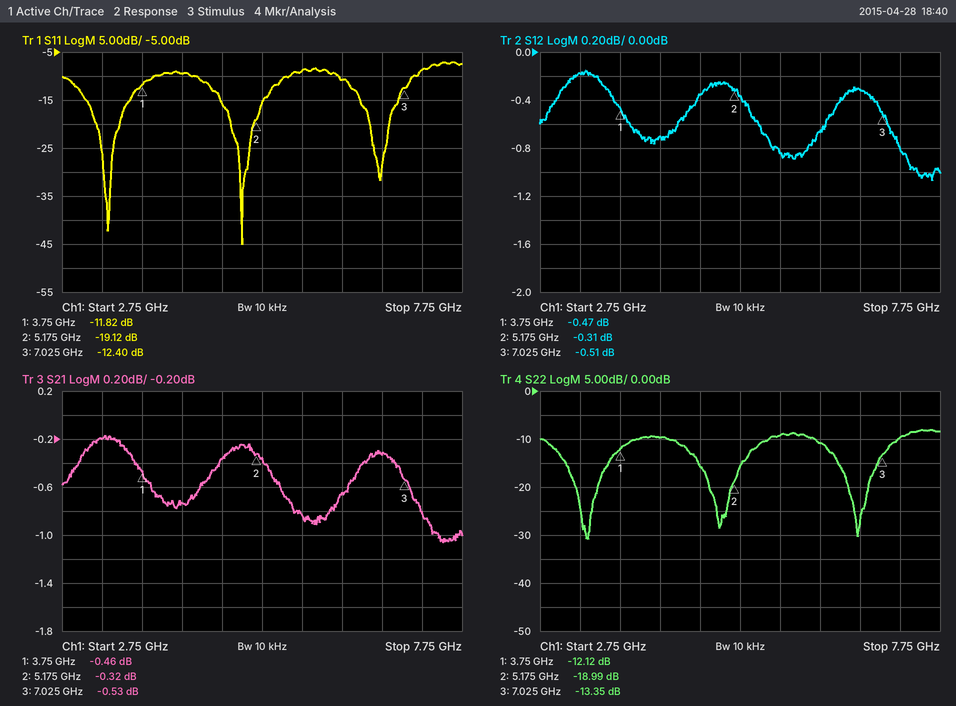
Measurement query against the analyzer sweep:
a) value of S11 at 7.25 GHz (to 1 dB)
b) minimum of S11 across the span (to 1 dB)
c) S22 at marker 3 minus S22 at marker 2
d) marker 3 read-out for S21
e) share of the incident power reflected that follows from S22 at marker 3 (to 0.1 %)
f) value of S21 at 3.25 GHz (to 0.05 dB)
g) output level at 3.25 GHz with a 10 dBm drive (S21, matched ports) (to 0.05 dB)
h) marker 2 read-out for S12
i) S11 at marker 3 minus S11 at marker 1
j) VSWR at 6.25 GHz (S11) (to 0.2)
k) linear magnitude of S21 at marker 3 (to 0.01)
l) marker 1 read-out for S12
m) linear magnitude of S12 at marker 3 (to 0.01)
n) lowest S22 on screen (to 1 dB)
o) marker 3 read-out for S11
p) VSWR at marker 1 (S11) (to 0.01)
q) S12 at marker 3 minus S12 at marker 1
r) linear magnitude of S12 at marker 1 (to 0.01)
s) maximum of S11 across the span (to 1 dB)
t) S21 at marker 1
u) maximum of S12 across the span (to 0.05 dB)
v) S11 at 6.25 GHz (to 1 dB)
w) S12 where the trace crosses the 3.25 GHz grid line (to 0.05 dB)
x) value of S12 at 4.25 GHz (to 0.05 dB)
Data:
-9 dB
-45 dB
5.64 dB
-0.53 dB
4.6 %
-0.20 dB
9.80 dBm
-0.31 dB
-0.58 dB
1.8
0.94
-0.47 dB
0.94
-31 dB
-12.40 dB
1.69
-0.04 dB
0.95
-7 dB
-0.46 dB
-0.15 dB
-11 dB
-0.20 dB
-0.70 dB
